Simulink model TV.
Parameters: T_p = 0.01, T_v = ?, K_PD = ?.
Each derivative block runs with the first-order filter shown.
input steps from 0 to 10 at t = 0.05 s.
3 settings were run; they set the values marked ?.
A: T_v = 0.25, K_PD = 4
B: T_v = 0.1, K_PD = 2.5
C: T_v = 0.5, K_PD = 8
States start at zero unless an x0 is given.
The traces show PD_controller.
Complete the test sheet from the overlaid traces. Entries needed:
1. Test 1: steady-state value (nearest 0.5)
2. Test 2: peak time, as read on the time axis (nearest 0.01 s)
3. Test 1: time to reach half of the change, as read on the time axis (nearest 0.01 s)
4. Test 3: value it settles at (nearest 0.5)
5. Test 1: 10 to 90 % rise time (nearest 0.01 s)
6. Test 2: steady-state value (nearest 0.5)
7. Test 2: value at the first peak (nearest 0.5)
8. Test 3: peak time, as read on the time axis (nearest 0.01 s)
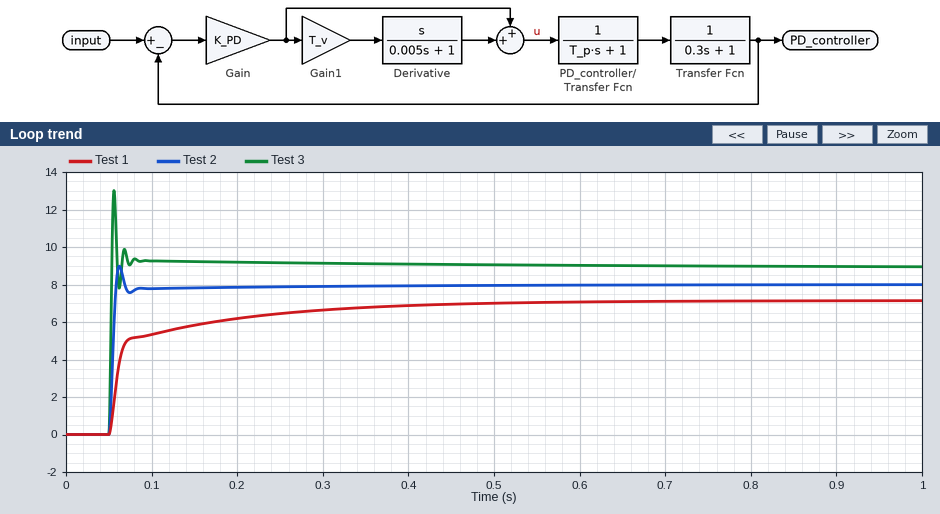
7.0
0.06 s
0.06 s
9.0
0.19 s
8.0
9.0
0.06 s
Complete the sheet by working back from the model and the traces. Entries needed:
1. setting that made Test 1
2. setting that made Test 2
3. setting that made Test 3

B
A
C
